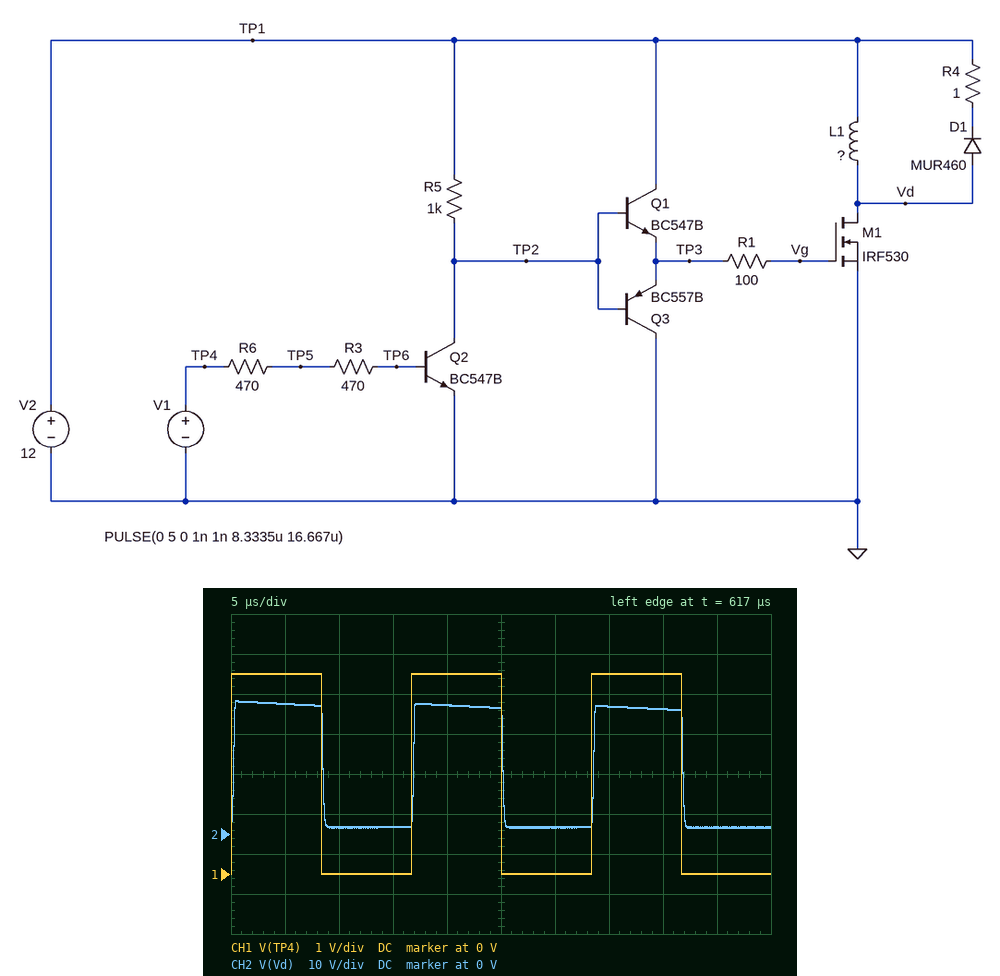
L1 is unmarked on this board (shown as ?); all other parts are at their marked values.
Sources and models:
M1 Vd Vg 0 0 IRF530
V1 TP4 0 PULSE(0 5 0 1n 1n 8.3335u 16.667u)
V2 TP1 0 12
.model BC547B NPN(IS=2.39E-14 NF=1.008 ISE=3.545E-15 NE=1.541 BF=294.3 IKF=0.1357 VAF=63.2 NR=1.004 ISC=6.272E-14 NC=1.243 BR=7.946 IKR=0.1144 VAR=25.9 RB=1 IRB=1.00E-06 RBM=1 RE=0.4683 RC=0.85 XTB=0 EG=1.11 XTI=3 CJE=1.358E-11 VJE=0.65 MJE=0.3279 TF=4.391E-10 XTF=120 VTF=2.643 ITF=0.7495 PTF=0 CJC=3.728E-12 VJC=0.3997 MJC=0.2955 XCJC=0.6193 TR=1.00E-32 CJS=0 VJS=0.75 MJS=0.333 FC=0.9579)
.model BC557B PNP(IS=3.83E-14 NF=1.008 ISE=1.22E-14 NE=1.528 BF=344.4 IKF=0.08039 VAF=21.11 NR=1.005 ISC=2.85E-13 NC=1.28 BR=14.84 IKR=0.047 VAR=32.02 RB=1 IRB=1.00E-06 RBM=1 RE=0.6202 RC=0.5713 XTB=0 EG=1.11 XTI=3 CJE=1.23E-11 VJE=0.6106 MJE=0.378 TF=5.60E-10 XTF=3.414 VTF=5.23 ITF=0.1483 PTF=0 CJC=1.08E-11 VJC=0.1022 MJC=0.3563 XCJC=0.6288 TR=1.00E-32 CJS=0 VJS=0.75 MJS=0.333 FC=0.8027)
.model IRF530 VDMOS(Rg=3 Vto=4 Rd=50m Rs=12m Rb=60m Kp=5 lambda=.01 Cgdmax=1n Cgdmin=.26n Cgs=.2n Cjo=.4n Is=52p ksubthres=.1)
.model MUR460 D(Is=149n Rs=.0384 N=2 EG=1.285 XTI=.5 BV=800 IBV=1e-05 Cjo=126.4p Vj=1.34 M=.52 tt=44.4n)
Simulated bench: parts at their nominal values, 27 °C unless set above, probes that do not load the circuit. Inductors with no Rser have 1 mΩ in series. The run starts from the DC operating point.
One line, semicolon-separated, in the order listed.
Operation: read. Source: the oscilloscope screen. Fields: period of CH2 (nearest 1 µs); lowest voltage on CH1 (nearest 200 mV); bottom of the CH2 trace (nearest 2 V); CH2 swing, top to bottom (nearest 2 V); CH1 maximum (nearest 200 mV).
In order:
17 µs; 0 V; 2 V; 32 V; 5.0 V
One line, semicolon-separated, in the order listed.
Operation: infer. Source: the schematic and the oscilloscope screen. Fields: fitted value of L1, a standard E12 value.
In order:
150 µH
